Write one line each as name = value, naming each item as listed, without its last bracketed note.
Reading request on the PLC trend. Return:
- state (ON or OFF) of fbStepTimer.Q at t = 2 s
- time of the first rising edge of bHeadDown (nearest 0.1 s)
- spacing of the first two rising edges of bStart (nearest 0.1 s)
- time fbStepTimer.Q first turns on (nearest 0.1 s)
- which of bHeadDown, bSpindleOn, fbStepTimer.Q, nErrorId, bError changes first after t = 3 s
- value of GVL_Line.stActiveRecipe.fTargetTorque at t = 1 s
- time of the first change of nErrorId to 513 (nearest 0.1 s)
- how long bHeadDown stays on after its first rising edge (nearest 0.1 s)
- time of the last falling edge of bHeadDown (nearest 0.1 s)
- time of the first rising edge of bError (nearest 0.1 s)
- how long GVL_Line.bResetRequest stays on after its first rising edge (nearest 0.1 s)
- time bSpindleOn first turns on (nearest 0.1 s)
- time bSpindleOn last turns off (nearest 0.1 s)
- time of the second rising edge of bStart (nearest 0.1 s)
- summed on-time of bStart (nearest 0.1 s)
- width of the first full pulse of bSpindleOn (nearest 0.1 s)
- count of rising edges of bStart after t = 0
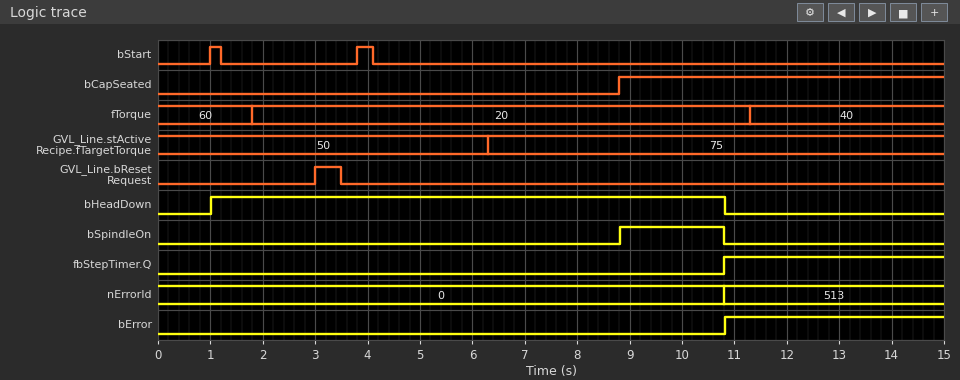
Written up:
state (ON or OFF) of fbStepTimer.Q at t = 2 s = OFF
time of the first rising edge of bHeadDown = 1.0 s
spacing of the first two rising edges of bStart = 2.8 s
time fbStepTimer.Q first turns on = 10.8 s
which of bHeadDown, bSpindleOn, fbStepTimer.Q, nErrorId, bError changes first after t = 3 s = bSpindleOn
value of GVL_Line.stActiveRecipe.fTargetTorque at t = 1 s = 50
time of the first change of nErrorId to 513 = 10.8 s
how long bHeadDown stays on after its first rising edge = 9.8 s
time of the last falling edge of bHeadDown = 10.8 s
time of the first rising edge of bError = 10.8 s
how long GVL_Line.bResetRequest stays on after its first rising edge = 0.5 s
time bSpindleOn first turns on = 8.8 s
time bSpindleOn last turns off = 10.8 s
time of the second rising edge of bStart = 3.8 s
summed on-time of bStart = 0.5 s
width of the first full pulse of bSpindleOn = 2.0 s
count of rising edges of bStart after t = 0 = 2
